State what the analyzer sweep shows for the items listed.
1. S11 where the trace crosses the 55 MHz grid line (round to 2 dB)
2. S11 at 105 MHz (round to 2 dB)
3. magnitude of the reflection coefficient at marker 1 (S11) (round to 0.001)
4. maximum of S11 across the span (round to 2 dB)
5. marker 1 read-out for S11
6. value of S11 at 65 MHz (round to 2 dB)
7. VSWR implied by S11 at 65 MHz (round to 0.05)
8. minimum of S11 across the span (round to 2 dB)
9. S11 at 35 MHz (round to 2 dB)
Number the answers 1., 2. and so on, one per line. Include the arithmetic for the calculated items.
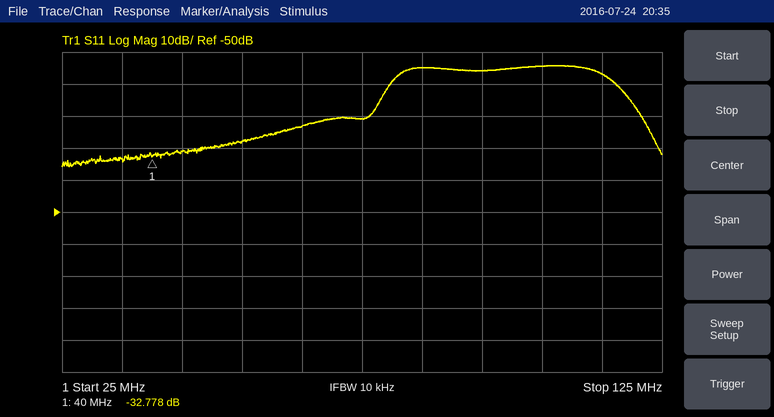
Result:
1. -28 dB
2. -4 dB
3. 10^(-32.778/20) ≈ 0.023
4. -4 dB
5. -32.778 dB
6. -24 dB
7. |Γ| = 10^(-24/20) = 0.0631; VSWR = (1 + 0.0631)/(1 − 0.0631) ≈ 1.13, so 1.15 to the nearest 0.05
8. -36 dB
9. -34 dB
